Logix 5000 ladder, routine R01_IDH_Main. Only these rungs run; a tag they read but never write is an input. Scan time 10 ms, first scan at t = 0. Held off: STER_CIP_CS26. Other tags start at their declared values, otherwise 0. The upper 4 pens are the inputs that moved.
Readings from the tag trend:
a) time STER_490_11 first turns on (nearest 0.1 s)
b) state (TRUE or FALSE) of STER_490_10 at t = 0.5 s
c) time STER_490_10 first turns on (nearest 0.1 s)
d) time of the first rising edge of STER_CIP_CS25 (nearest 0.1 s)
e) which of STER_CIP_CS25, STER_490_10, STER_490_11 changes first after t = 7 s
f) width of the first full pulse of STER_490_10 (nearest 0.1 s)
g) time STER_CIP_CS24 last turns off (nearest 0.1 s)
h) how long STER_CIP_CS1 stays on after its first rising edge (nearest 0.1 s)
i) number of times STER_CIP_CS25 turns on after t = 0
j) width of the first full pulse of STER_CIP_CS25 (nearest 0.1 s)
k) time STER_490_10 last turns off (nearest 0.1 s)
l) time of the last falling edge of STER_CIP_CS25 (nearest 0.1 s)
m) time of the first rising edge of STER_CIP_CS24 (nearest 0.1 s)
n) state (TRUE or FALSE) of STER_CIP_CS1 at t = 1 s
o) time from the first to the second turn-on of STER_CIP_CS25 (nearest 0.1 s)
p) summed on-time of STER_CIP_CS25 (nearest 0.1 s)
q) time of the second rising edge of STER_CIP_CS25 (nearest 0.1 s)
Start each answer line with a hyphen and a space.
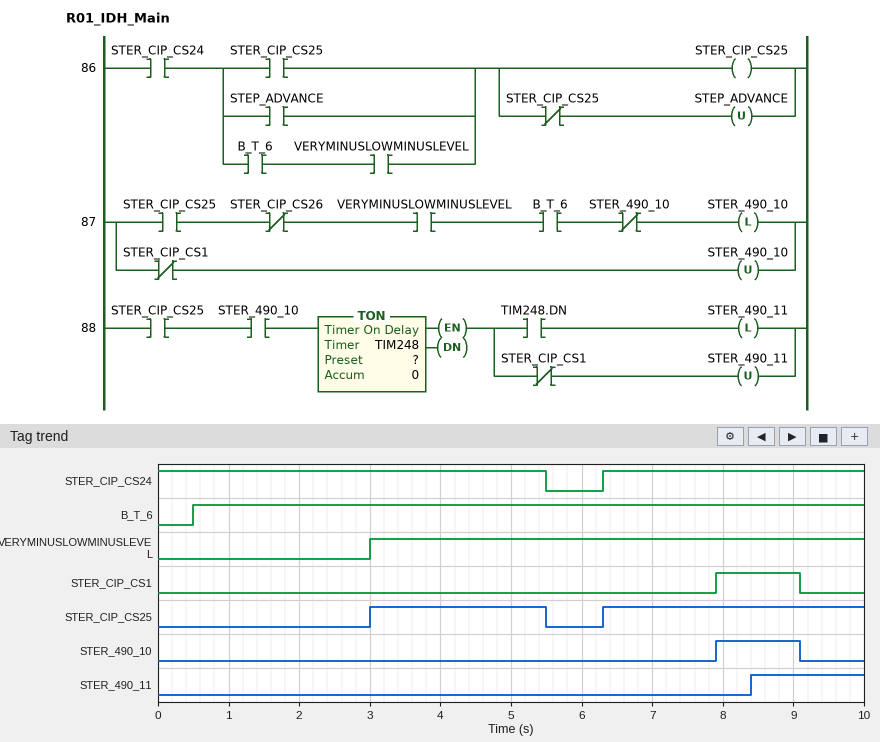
- 8.4 s
- FALSE
- 7.9 s
- 3.0 s
- STER_490_10
- 1.2 s
- 5.5 s
- 1.2 s
- 2
- 2.5 s
- 9.1 s
- 5.5 s
- 6.3 s
- FALSE
- 3.3 s
- 6.2 s
- 6.3 s
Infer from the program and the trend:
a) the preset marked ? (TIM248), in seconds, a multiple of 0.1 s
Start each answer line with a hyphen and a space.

- 0.5 s
